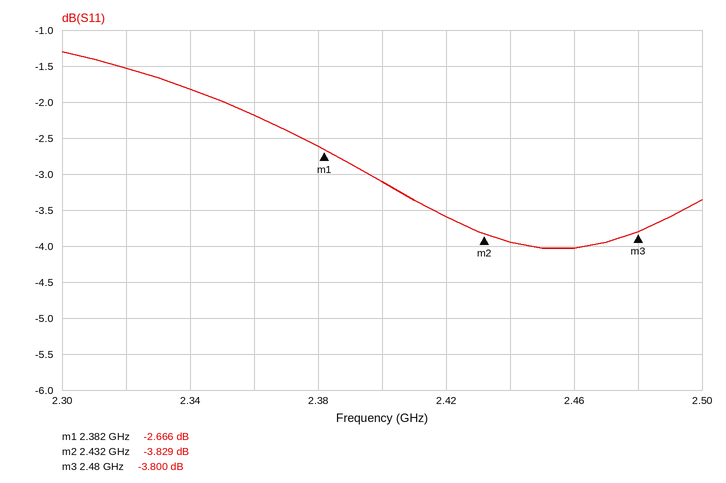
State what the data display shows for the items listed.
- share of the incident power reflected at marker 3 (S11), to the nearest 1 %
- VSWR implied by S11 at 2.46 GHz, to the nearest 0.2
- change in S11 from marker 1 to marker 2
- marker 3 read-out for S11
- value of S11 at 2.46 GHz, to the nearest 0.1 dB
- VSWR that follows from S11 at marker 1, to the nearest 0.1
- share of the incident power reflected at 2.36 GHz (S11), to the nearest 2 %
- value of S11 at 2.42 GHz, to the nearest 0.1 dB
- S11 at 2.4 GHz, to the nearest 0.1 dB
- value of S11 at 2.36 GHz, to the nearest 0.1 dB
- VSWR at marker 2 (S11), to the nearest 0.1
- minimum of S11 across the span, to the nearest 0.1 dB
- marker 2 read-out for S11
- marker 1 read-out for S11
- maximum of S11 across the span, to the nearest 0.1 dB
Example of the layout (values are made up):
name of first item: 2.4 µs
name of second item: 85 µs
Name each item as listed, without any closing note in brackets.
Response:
share of the incident power reflected at marker 3 (S11), to the nearest 1 %: 42 %
VSWR implied by S11 at 2.46 GHz, to the nearest 0.2: 4.4
change in S11 from marker 1 to marker 2: -1.163 dB
marker 3 read-out for S11: -3.800 dB
value of S11 at 2.46 GHz, to the nearest 0.1 dB: -4.0 dB
VSWR that follows from S11 at marker 1, to the nearest 0.1: 6.6
share of the incident power reflected at 2.36 GHz (S11), to the nearest 2 %: 60 %
value of S11 at 2.42 GHz, to the nearest 0.1 dB: -3.6 dB
S11 at 2.4 GHz, to the nearest 0.1 dB: -3.1 dB
value of S11 at 2.36 GHz, to the nearest 0.1 dB: -2.2 dB
VSWR at marker 2 (S11), to the nearest 0.1: 4.6
minimum of S11 across the span, to the nearest 0.1 dB: -4.0 dB
marker 2 read-out for S11: -3.829 dB
marker 1 read-out for S11: -2.666 dB
maximum of S11 across the span, to the nearest 0.1 dB: -1.3 dB
